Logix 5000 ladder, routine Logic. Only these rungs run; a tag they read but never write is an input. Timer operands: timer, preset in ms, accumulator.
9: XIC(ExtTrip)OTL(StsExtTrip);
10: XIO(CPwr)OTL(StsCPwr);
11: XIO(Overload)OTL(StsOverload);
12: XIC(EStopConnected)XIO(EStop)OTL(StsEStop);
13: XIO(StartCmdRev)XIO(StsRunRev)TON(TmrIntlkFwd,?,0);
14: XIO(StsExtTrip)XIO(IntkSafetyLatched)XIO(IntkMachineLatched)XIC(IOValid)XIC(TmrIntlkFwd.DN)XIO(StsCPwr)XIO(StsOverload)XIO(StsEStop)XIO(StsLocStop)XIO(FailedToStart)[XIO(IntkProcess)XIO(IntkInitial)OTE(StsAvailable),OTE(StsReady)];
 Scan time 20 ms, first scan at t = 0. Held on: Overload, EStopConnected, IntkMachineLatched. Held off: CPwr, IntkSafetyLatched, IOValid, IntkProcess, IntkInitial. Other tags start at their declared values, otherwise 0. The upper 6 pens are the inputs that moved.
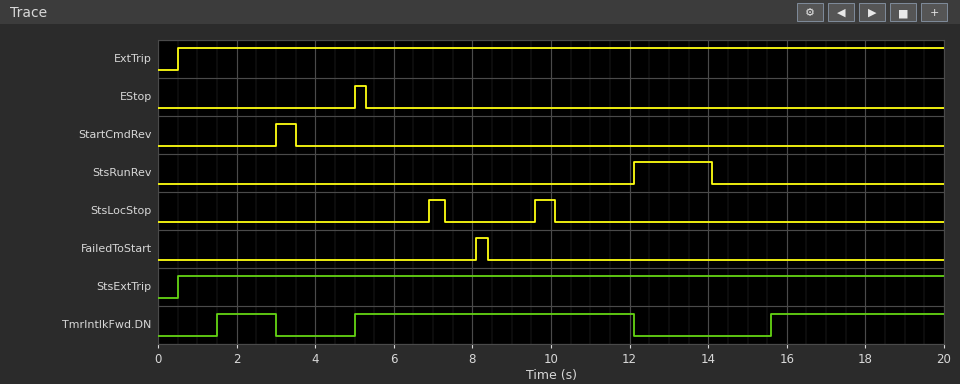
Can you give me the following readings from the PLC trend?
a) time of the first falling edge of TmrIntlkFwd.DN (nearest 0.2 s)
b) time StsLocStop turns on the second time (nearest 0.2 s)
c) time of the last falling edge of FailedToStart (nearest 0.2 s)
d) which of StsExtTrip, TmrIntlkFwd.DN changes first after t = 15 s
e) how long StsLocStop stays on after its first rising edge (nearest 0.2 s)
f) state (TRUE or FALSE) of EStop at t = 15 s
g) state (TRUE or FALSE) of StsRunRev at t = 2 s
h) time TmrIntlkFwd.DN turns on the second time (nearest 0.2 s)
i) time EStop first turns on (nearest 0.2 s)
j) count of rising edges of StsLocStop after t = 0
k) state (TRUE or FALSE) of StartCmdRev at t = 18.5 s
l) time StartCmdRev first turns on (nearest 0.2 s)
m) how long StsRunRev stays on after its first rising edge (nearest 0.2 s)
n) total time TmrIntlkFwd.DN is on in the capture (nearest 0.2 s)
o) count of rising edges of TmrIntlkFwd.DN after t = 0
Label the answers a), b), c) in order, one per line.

a) 3.0 s
b) 9.6 s
c) 8.4 s
d) TmrIntlkFwd.DN
e) 0.4 s
f) FALSE
g) FALSE
h) 5.0 s
i) 5.0 s
j) 2
k) FALSE
l) 3.0 s
m) 2.0 s
n) 13.0 s
o) 3
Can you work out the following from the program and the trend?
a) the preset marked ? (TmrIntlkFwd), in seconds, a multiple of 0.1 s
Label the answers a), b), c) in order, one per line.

a) 1.5 s
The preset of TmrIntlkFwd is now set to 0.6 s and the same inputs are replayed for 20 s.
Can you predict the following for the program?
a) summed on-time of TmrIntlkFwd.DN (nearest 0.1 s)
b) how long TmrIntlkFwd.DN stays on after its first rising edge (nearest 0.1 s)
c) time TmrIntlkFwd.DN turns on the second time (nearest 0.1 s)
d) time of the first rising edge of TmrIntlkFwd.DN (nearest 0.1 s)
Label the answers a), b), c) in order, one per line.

a) 15.7 s
b) 2.4 s
c) 4.1 s
d) 0.6 s
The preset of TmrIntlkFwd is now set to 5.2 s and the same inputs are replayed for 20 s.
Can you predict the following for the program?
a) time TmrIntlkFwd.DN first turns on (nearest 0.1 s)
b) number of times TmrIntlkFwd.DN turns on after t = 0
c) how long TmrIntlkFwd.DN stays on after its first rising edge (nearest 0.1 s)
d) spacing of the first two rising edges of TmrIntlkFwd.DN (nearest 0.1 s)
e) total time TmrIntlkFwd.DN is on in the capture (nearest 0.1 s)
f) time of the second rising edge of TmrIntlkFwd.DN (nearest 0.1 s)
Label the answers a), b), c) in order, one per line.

a) 8.7 s
b) 2
c) 3.4 s
d) 10.6 s
e) 4.1 s
f) 19.3 s
